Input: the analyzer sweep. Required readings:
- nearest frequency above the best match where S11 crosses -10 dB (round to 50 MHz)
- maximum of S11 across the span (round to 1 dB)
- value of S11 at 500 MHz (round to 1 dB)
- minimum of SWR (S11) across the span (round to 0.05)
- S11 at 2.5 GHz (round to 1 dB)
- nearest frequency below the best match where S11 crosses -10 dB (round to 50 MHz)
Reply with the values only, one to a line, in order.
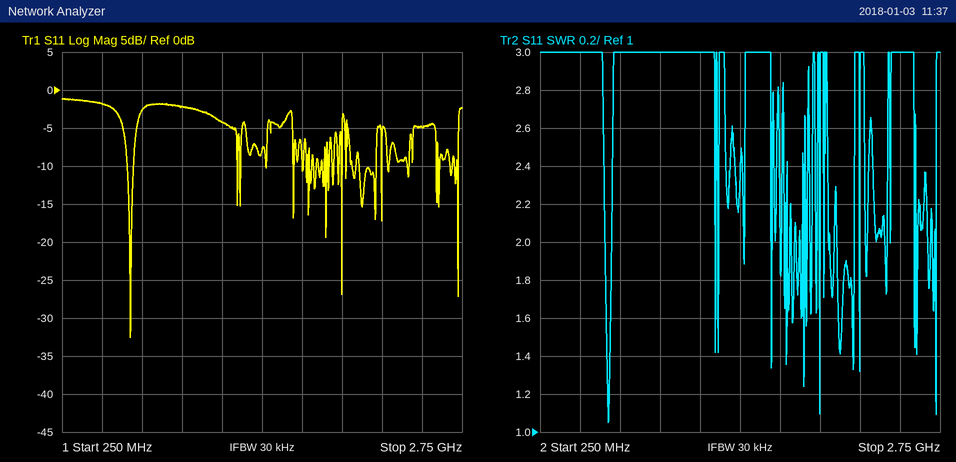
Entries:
700 MHz
-1 dB
-2 dB
1.05
-5 dB
650 MHz
